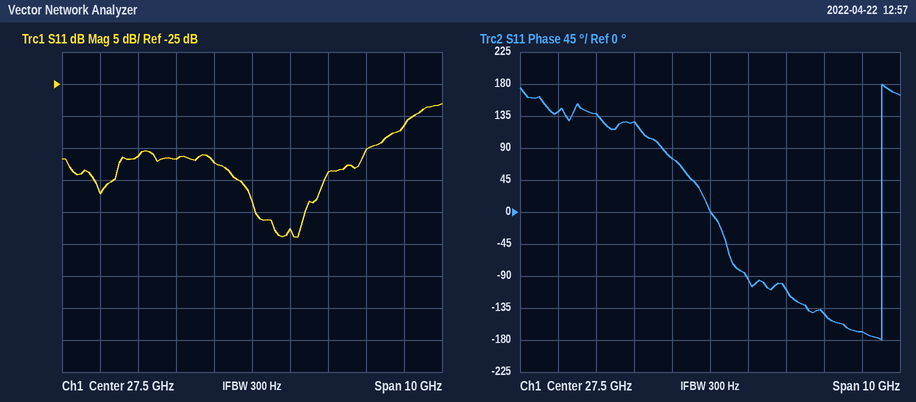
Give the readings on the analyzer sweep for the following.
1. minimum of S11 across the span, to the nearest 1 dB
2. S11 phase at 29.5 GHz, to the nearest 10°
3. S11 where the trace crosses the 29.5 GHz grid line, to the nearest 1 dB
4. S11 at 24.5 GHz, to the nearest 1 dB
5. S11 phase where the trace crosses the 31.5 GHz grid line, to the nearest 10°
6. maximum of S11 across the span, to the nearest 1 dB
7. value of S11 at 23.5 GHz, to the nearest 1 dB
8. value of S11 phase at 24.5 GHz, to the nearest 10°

-49 dB
-110°
-39 dB
-36 dB
-170°
-28 dB
-42 dB
140°
